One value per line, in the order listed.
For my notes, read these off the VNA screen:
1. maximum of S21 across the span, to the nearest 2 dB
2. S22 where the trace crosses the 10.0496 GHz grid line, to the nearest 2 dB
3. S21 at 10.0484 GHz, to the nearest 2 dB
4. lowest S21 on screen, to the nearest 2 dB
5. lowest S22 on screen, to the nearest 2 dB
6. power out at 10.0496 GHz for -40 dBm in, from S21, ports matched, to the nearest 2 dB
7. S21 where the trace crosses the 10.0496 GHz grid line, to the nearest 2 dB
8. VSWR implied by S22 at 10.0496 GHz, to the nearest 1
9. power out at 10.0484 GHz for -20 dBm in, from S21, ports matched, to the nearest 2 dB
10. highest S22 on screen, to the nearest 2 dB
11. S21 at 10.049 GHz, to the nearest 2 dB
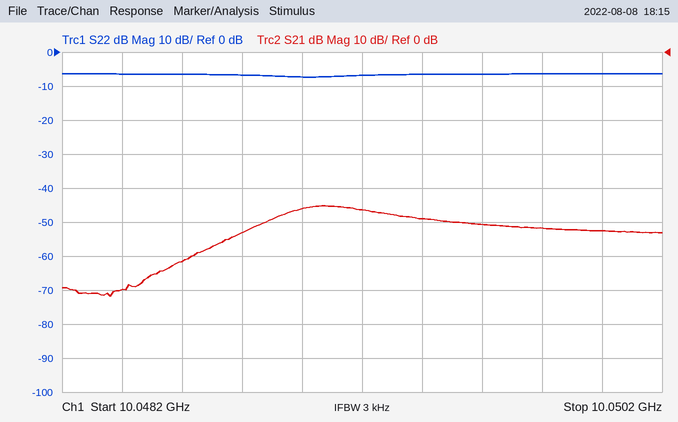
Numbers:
-46 dB
-6 dB
-70 dB
-72 dB
-8 dB
-90 dBm
-50 dB
3
-90 dBm
-6 dB
-46 dB
